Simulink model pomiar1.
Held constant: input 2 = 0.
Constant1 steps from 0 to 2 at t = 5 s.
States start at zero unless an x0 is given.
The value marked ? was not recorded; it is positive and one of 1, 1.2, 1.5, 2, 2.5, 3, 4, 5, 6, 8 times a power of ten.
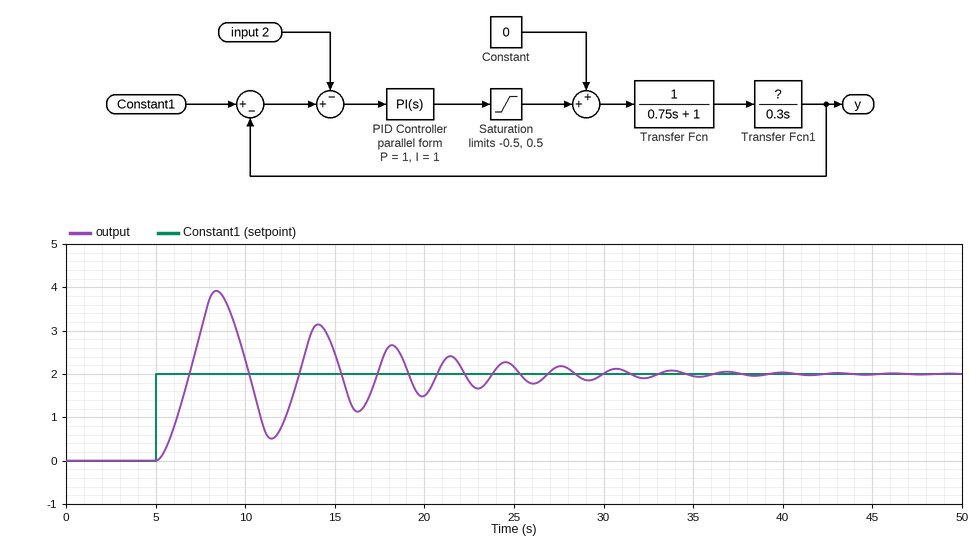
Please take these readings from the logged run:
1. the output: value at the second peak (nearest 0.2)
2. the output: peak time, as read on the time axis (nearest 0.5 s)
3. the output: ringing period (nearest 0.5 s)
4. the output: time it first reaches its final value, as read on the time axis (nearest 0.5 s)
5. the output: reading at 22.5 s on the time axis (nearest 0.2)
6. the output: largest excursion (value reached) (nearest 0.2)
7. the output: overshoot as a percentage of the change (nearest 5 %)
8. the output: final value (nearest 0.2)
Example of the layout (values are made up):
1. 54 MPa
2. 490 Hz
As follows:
1. 3.2
2. 8.5 s
3. 5.5 s
4. 7.0 s
5. 1.8
6. 4.0
7. 95 %
8. 2.0
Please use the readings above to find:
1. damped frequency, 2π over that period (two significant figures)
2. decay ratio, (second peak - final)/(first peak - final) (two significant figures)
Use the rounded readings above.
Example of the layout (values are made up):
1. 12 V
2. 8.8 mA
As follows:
1. 1.1 rad/s
2. 0.60
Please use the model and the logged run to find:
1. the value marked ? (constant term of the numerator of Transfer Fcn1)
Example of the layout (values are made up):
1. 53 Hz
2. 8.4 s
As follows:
1. 1
